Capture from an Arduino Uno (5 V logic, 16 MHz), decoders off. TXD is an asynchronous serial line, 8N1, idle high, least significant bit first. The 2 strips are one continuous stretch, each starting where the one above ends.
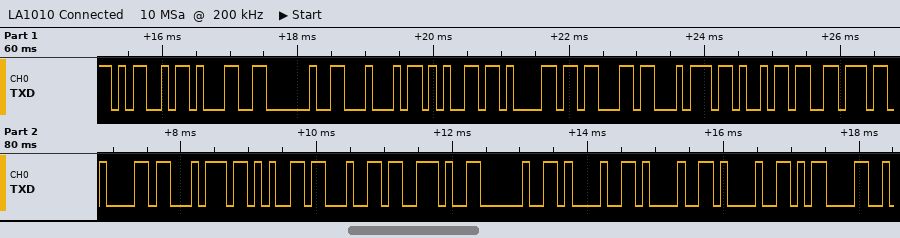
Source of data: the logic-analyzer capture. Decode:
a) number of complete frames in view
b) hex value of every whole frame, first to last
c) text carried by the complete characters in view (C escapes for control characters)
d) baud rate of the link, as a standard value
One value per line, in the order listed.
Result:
20
0x4D 0x31 0x20 0x44 0x65 0x61 0x63 0x74 0x69 0x76 0x61 0x74 0x65 0x64 0x2E 0x20 0x21 0x21 0x21 0x0D
"M1 Deactivated. !!!\r"
9600 baud
